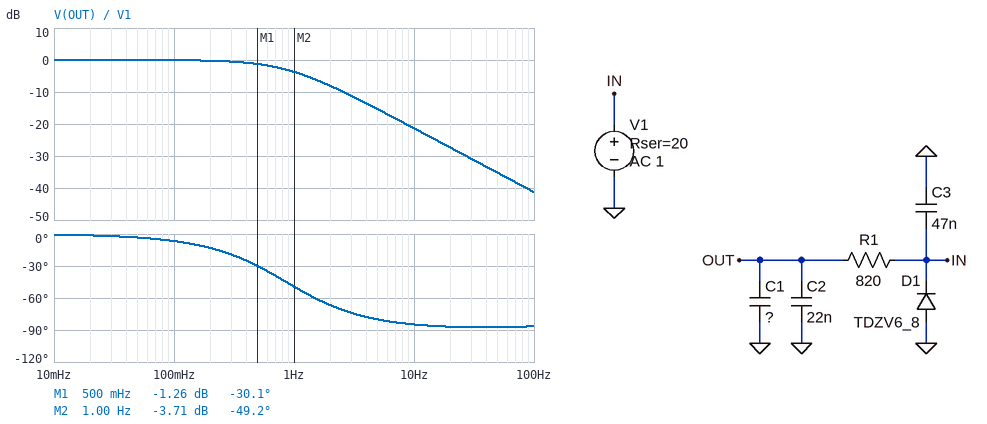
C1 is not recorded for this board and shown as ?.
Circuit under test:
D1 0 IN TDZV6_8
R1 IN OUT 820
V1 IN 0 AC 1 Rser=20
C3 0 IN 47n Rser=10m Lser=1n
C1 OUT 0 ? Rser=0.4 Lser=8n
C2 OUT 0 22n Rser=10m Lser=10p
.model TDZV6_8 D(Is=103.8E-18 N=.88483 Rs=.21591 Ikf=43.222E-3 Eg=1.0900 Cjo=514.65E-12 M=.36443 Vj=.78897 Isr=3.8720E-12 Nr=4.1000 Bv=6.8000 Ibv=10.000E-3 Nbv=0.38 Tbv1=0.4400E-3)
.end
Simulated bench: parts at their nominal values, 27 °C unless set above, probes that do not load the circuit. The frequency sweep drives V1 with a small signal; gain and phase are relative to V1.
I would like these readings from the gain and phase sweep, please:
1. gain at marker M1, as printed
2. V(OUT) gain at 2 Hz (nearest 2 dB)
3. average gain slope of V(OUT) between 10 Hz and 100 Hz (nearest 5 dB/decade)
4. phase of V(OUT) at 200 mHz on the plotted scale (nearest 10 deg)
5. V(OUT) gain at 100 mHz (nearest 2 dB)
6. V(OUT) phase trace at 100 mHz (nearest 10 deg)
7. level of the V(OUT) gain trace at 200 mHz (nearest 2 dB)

-1.26 dB
-8 dB
-20 dB/decade
-10 deg
0 dB
-10 deg
0 dB
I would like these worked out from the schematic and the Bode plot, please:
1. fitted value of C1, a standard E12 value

220 µF
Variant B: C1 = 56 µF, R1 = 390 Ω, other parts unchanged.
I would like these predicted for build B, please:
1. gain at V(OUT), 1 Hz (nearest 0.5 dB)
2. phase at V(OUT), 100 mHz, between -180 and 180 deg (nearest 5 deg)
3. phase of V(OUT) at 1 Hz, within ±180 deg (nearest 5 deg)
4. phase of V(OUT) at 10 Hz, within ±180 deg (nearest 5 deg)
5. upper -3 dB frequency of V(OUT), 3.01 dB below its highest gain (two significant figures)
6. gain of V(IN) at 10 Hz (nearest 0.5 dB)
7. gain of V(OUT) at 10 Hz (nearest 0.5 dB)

0 dB
0 deg
-10 deg
-55 deg
6.9 Hz
-0.5 dB
-5.0 dB
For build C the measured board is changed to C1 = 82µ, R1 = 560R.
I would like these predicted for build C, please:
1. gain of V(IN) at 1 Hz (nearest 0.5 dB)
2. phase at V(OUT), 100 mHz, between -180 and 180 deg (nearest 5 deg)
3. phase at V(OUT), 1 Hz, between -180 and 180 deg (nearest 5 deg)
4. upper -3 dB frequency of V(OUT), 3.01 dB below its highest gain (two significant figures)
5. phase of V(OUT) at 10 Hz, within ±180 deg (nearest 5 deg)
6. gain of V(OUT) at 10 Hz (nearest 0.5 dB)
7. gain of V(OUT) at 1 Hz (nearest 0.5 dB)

0 dB
0 deg
-15 deg
3.3 Hz
-70 deg
-10.0 dB
-0.5 dB
